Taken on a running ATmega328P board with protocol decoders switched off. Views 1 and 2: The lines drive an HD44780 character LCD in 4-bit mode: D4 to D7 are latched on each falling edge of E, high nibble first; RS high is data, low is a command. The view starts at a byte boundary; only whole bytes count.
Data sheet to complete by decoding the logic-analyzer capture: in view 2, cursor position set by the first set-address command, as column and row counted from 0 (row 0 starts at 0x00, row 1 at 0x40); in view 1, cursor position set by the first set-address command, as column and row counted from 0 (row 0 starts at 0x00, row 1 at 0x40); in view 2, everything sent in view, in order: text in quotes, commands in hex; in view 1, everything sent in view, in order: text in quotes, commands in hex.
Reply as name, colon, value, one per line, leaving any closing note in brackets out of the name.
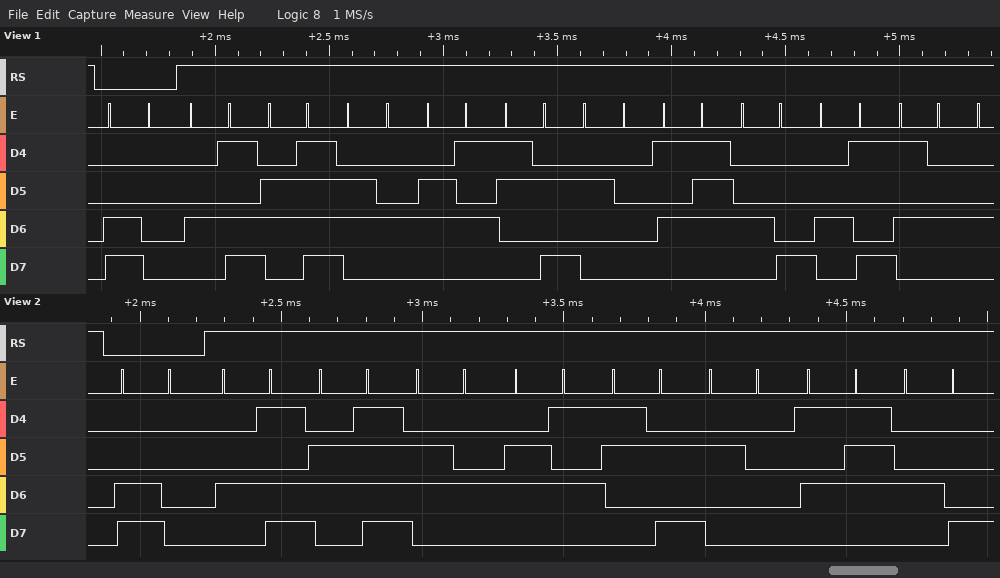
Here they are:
in view 2, cursor position set by the first set-address command, as column and row counted from 0: column 0, row 1
in view 1, cursor position set by the first set-address command, as column and row counted from 0: column 0, row 1
in view 2, everything sent in view, in order: text in quotes, commands in hex: 0xC0 "Mode: WH"
in view 1, everything sent in view, in order: text in quotes, commands in hex: 0xC0 "Mode: WHIT"
